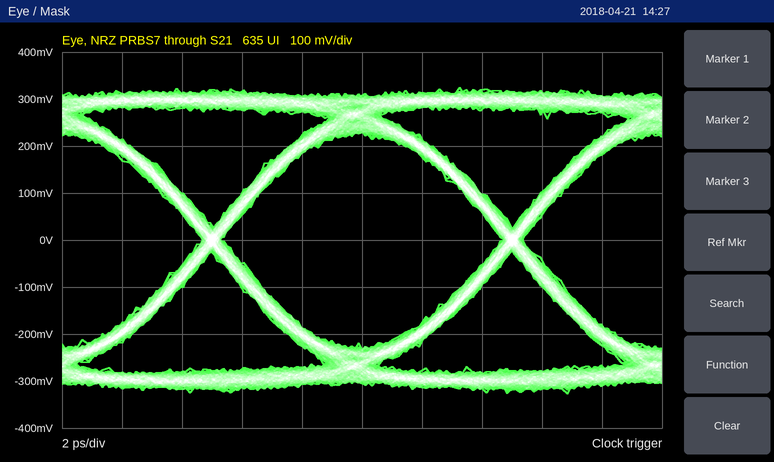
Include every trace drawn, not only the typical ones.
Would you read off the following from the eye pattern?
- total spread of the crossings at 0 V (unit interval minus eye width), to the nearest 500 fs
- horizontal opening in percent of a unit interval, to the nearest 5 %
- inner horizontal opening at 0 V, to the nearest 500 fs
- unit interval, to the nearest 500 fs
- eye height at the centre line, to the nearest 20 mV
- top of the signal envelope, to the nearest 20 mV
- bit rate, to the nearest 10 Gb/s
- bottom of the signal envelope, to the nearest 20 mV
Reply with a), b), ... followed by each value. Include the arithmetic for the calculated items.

a) 500 fs
b) 9.5 ps / 10.0 ps ≈ 95 %
c) 9.5 ps
d) 10.0 ps
e) 460 mV
f) 320 mV
g) 100 Gb/s
h) -320 mV
